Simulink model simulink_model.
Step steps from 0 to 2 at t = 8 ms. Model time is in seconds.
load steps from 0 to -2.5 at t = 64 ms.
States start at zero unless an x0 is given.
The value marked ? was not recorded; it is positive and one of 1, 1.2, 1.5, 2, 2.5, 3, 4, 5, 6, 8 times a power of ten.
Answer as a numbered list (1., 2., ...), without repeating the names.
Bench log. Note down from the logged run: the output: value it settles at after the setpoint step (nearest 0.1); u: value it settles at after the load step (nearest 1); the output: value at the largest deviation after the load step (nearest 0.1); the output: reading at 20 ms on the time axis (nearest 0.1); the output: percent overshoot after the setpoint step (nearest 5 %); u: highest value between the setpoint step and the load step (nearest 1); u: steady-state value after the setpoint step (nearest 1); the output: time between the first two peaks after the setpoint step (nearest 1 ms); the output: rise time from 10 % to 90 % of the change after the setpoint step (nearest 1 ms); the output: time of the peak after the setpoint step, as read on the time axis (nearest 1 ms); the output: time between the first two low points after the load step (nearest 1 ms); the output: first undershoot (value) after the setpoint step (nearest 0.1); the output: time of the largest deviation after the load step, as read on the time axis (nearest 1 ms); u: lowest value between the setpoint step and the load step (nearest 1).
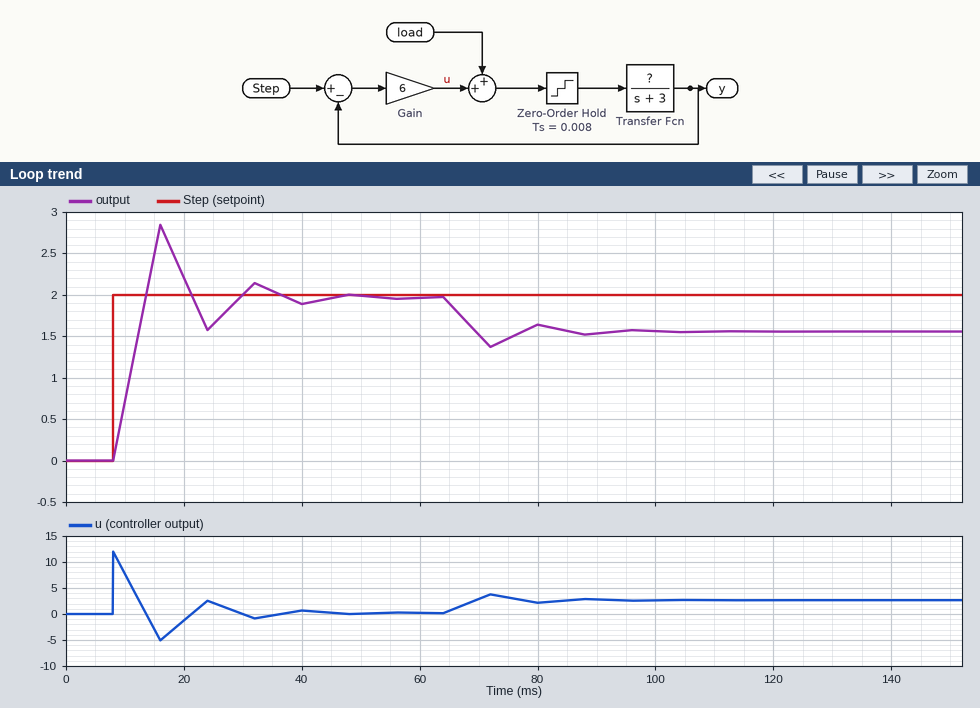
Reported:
1. 2.0
2. 3
3. 1.4
4. 2.2
5. 45 %
6. 12
7. 0
8. 16 ms
9. 4 ms
10. 16 ms
11. 16 ms
12. 1.6
13. 72 ms
14. -5
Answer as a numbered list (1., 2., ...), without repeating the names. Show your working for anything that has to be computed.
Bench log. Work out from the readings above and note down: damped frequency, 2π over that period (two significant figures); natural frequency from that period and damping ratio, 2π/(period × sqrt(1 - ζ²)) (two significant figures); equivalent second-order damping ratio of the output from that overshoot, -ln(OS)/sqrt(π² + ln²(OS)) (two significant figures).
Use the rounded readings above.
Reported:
1. 2π / 16 = 0.39 rad/ms
2. 2π / (16 × sqrt(1 - 0.25²)) = 0.41 rad/ms
3. ln(0.45) = -0.799; 0.799 / sqrt(9.870 + 0.638) = 0.25
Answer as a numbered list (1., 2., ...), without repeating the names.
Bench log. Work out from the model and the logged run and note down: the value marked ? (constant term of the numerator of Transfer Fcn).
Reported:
1. 30
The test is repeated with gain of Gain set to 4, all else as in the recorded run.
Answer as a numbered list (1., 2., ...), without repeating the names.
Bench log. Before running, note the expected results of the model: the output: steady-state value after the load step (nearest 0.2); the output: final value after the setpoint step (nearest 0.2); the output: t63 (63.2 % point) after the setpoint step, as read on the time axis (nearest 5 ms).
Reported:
1. 1.4
2. 2.0
3. 15 ms
